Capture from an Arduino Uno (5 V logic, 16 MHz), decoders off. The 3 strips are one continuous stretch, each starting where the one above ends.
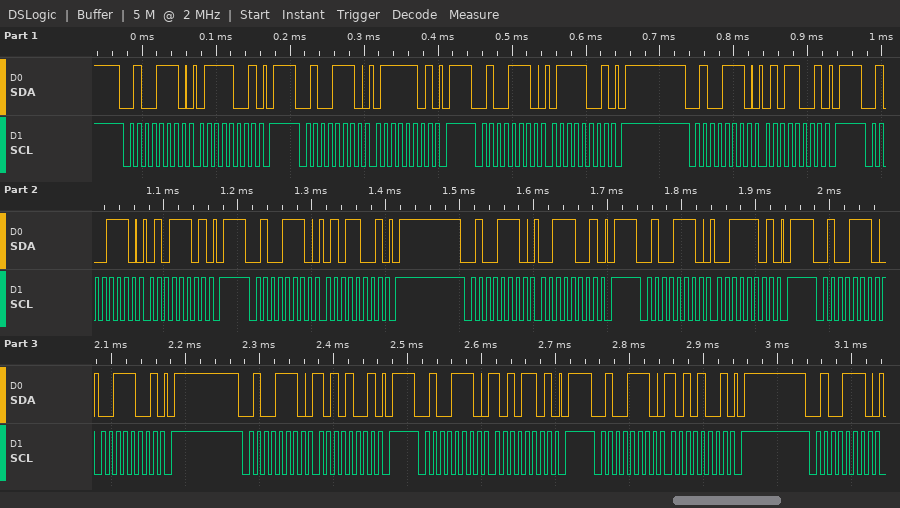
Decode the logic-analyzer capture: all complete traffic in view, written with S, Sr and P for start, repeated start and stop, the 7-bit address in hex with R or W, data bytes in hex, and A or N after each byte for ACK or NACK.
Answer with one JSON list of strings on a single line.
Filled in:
["S 27W A 79 A P S 27W A 7D A P S 27W A 79 A P S 27W A 59 A P S 27W A 5D A P S 27W A 59 A P S 27W A 39 A P S 27W A 3D A P S 27W A 39 A P S 27W A A9 A P S 27W A AD A P S 27W A A9 A P S 27W A"]
